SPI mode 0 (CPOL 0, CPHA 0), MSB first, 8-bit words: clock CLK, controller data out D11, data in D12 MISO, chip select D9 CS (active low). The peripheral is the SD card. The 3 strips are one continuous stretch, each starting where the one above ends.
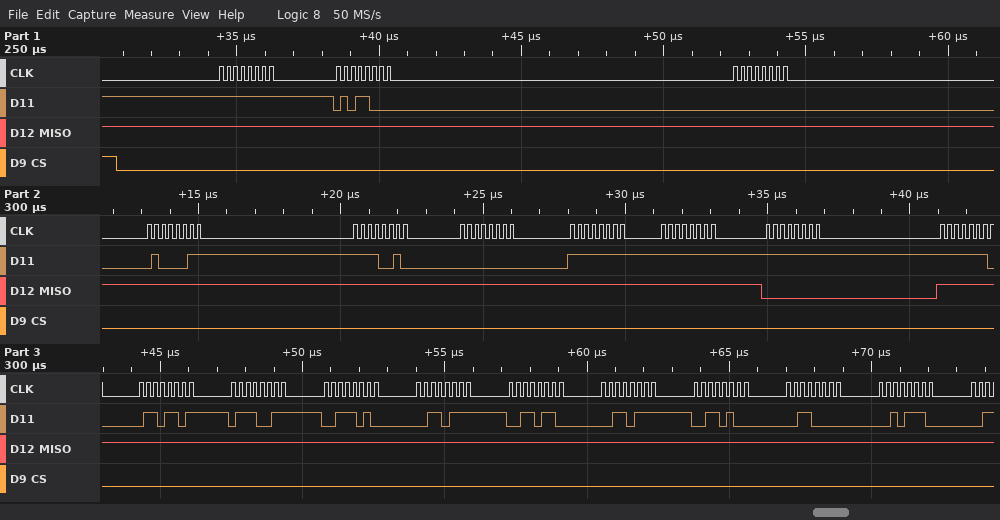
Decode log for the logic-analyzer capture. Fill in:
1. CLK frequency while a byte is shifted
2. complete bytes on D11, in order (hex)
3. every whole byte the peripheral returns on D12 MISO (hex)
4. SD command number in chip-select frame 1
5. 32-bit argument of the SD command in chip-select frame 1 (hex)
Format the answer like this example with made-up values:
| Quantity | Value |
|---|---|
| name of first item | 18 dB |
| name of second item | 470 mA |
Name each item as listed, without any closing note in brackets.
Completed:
| Quantity | Value |
|---|---|
| CLK frequency while a byte is shifted | 4 MHz |
| complete bytes on D11, in order | 0xFF 0x58 0x00 0x43 0xF2 0x00 0xFF 0xFF 0xFF 0xFE 0x6D 0x73 0x3A 0x37 0x36 0x37 0x34 0x30 0x2E |
| every whole byte the peripheral returns on D12 MISO | 0xFF 0xFF 0xFF 0xFF 0xFF 0xFF 0xFF 0xFF 0x00 0xFF 0xFF 0xFF 0xFF 0xFF 0xFF 0xFF 0xFF 0xFF 0xFF |
| SD command number in chip-select frame 1 | CMD24 |
| 32-bit argument of the SD command in chip-select frame 1 | 0x0043F200 |
